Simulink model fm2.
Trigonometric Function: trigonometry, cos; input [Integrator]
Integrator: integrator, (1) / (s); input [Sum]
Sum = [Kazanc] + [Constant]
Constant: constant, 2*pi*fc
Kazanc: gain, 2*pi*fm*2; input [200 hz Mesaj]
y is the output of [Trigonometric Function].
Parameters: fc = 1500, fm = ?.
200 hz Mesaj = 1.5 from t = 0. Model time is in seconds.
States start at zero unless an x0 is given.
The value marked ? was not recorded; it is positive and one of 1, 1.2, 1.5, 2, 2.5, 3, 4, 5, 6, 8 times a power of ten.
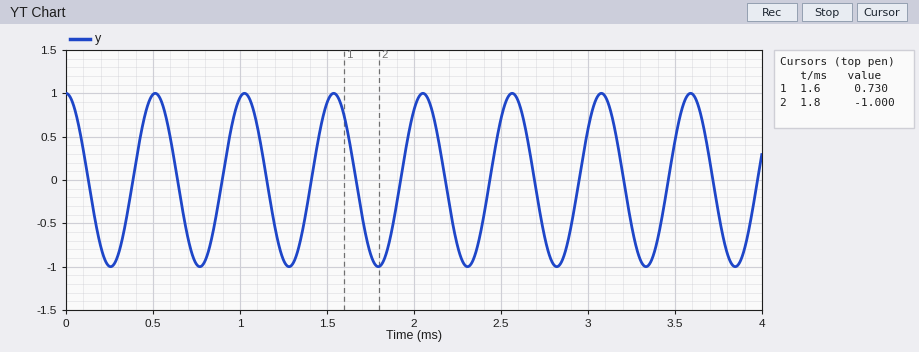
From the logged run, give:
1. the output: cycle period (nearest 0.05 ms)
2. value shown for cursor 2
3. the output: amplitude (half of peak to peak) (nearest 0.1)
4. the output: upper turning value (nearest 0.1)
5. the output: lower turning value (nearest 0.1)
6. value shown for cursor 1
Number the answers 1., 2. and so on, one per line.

1. 0.50 ms
2. -1.000
3. 1.0
4. 1.0
5. -1.0
6. 0.730
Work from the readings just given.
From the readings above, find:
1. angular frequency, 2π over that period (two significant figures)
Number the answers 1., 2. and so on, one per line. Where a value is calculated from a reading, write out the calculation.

1. 2π / 0.5 = 13 rad/ms
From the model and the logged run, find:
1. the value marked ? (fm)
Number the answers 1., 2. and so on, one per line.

1. 150
